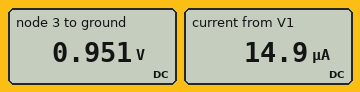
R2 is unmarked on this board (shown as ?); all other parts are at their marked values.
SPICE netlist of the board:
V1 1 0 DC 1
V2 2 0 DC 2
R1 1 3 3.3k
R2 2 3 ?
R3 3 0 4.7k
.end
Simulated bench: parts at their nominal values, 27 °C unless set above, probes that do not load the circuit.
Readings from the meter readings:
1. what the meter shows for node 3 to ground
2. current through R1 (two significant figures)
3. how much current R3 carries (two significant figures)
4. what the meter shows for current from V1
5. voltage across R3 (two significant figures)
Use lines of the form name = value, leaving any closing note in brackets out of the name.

what the meter shows for node 3 to ground = 0.951 V
current through R1 = 15 µA
how much current R3 carries = 200 µA
what the meter shows for current from V1 = 14.9 µA
voltage across R3 = 950 mV
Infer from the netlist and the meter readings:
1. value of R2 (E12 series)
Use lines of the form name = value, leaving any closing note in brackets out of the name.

value of R2 = 5.6 kΩ
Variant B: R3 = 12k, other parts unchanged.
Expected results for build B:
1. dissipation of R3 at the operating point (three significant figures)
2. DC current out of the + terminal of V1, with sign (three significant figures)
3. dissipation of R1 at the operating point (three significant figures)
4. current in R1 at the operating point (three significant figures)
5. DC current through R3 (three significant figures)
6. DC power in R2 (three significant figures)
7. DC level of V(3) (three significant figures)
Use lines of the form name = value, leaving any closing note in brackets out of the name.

dissipation of R3 at the operating point = 114 µW
DC current out of the + terminal of V1, with sign = -51.1 µA
dissipation of R1 at the operating point = 8.61 µW
current in R1 at the operating point = 51.1 µA
DC current through R3 = 97.4 µA
DC power in R2 = 123 µW
DC level of V(3) = 1.17 V
